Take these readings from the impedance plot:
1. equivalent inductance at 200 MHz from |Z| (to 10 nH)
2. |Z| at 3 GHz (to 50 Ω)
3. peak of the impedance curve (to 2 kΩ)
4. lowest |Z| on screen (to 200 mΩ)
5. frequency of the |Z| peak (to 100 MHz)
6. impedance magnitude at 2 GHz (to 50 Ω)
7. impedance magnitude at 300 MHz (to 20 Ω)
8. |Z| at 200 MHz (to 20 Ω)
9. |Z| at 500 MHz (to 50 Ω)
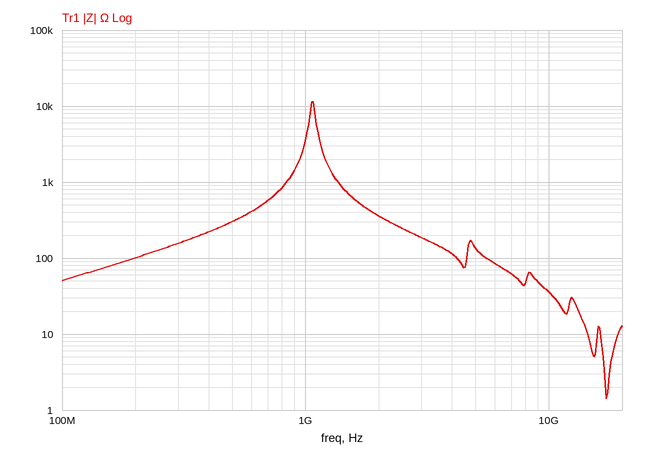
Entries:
80 nH
200 Ω
12 kΩ
1.4 Ω
1.1 GHz
350 Ω
160 Ω
100 Ω
300 Ω
